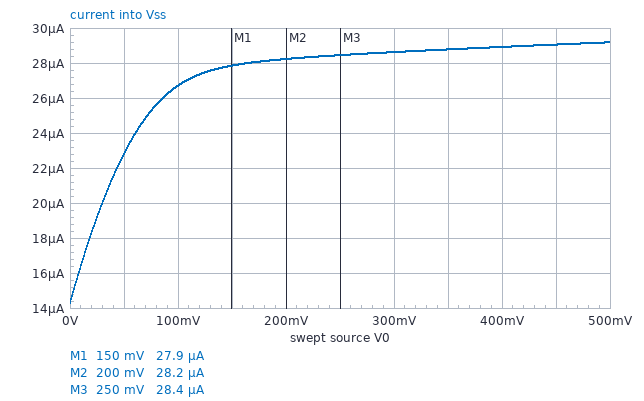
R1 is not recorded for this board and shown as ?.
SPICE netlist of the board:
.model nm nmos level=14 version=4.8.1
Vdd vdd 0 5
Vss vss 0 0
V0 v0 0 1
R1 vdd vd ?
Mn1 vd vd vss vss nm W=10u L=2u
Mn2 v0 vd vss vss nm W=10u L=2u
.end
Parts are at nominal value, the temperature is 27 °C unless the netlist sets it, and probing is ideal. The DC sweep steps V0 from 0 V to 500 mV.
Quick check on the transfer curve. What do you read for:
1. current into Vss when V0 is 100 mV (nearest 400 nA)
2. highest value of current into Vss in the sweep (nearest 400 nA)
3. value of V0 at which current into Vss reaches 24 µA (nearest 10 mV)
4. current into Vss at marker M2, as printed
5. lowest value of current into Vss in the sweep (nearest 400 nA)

26.8 µA
29.2 µA
60 mV
28.2 µA
14.4 µA
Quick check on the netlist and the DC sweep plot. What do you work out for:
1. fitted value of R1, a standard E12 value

330 kΩ
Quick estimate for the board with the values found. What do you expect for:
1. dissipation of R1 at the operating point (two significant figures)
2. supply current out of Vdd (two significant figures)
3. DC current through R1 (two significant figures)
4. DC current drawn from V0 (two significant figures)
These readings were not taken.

67 µW
14 µA
14 µA
16 µA
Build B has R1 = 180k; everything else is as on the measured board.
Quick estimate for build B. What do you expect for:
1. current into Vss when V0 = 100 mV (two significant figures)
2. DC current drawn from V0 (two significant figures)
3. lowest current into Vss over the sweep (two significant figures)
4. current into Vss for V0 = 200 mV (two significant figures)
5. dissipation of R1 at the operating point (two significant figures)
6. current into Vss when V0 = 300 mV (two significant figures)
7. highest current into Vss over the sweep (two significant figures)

47 µA
29 µA
26 µA
51 µA
120 µW
52 µA
53 µA
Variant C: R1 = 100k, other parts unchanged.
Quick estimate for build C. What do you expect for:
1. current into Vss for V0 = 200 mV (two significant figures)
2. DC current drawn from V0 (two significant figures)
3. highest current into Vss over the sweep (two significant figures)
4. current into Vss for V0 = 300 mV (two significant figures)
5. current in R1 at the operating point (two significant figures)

90 µA
50 µA
94 µA
92 µA
46 µA
